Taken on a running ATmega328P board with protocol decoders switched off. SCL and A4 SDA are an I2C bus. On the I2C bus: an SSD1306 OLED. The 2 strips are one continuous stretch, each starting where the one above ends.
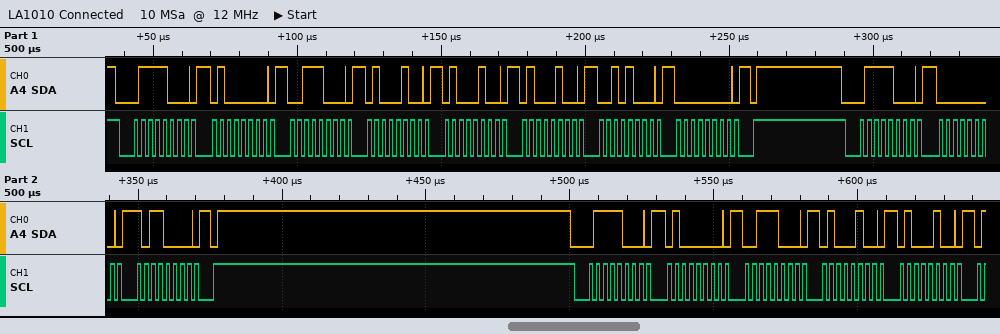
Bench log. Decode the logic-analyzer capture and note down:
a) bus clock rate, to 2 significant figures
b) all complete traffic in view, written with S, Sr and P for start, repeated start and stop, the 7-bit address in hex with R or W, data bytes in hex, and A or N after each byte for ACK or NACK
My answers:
400 kHz
S 3CW A 40 A 38 A 44 A 44 A 44 A 28 A 00 A P S 3CW A 00 A B0 A P S 3CW A 40 A 38 A 44 A 44 A
